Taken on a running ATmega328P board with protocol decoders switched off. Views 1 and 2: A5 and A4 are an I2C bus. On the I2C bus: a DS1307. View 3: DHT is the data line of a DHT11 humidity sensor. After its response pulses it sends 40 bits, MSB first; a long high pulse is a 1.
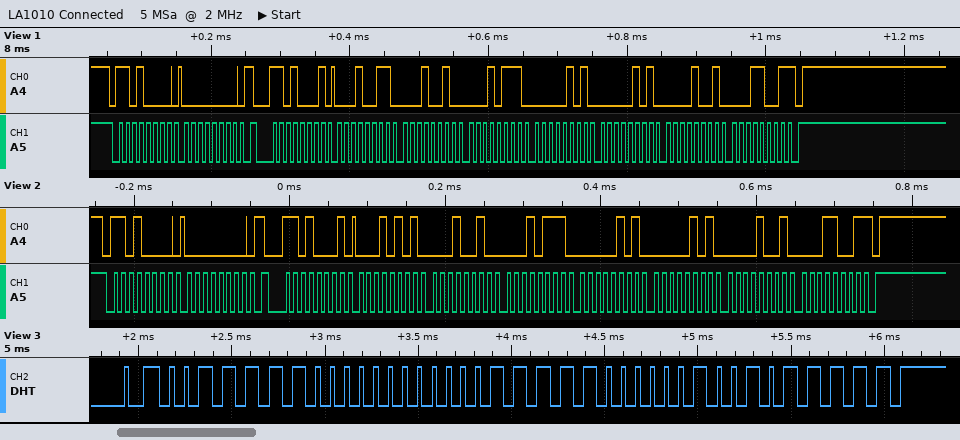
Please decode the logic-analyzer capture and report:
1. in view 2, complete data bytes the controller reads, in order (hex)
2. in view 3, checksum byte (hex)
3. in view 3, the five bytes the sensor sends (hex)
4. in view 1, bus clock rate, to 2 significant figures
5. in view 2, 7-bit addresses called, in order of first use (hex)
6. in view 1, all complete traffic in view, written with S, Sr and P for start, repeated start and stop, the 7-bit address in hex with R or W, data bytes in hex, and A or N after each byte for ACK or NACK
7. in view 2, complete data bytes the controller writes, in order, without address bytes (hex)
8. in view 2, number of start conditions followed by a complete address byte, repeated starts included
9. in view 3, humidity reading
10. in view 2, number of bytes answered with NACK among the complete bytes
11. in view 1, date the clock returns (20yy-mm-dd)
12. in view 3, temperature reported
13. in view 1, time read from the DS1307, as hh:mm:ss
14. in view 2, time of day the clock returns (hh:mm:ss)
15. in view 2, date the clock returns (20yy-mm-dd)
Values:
15 12 17 05 05 09 19
0x5F
3E 00 1F 02 5F
100 kHz
0x68
S 68W A 00 A Sr 68R A 13 A 12 A 17 A 05 A 05 A 09 A 19 N P
00
2
62 %
1
2019-09-05
31.2 °C
17:12:13
17:12:15
2019-09-05
